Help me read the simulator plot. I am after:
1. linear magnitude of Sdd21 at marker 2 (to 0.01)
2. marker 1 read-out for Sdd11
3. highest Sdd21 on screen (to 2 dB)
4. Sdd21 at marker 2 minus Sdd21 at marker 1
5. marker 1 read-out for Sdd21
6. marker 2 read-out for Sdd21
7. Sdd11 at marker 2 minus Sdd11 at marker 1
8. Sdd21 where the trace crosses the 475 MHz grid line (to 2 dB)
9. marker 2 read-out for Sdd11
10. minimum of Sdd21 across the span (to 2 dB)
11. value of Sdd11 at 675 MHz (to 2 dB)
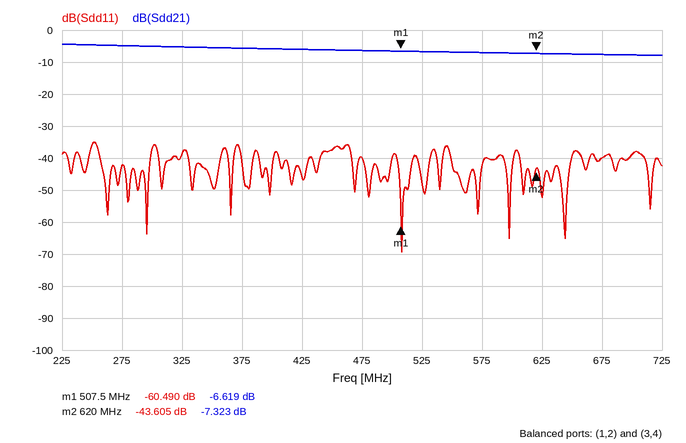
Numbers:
0.43
-60.490 dB
-4 dB
-0.704 dB
-6.619 dB
-7.323 dB
16.885 dB
-6 dB
-43.605 dB
-8 dB
-40 dB
